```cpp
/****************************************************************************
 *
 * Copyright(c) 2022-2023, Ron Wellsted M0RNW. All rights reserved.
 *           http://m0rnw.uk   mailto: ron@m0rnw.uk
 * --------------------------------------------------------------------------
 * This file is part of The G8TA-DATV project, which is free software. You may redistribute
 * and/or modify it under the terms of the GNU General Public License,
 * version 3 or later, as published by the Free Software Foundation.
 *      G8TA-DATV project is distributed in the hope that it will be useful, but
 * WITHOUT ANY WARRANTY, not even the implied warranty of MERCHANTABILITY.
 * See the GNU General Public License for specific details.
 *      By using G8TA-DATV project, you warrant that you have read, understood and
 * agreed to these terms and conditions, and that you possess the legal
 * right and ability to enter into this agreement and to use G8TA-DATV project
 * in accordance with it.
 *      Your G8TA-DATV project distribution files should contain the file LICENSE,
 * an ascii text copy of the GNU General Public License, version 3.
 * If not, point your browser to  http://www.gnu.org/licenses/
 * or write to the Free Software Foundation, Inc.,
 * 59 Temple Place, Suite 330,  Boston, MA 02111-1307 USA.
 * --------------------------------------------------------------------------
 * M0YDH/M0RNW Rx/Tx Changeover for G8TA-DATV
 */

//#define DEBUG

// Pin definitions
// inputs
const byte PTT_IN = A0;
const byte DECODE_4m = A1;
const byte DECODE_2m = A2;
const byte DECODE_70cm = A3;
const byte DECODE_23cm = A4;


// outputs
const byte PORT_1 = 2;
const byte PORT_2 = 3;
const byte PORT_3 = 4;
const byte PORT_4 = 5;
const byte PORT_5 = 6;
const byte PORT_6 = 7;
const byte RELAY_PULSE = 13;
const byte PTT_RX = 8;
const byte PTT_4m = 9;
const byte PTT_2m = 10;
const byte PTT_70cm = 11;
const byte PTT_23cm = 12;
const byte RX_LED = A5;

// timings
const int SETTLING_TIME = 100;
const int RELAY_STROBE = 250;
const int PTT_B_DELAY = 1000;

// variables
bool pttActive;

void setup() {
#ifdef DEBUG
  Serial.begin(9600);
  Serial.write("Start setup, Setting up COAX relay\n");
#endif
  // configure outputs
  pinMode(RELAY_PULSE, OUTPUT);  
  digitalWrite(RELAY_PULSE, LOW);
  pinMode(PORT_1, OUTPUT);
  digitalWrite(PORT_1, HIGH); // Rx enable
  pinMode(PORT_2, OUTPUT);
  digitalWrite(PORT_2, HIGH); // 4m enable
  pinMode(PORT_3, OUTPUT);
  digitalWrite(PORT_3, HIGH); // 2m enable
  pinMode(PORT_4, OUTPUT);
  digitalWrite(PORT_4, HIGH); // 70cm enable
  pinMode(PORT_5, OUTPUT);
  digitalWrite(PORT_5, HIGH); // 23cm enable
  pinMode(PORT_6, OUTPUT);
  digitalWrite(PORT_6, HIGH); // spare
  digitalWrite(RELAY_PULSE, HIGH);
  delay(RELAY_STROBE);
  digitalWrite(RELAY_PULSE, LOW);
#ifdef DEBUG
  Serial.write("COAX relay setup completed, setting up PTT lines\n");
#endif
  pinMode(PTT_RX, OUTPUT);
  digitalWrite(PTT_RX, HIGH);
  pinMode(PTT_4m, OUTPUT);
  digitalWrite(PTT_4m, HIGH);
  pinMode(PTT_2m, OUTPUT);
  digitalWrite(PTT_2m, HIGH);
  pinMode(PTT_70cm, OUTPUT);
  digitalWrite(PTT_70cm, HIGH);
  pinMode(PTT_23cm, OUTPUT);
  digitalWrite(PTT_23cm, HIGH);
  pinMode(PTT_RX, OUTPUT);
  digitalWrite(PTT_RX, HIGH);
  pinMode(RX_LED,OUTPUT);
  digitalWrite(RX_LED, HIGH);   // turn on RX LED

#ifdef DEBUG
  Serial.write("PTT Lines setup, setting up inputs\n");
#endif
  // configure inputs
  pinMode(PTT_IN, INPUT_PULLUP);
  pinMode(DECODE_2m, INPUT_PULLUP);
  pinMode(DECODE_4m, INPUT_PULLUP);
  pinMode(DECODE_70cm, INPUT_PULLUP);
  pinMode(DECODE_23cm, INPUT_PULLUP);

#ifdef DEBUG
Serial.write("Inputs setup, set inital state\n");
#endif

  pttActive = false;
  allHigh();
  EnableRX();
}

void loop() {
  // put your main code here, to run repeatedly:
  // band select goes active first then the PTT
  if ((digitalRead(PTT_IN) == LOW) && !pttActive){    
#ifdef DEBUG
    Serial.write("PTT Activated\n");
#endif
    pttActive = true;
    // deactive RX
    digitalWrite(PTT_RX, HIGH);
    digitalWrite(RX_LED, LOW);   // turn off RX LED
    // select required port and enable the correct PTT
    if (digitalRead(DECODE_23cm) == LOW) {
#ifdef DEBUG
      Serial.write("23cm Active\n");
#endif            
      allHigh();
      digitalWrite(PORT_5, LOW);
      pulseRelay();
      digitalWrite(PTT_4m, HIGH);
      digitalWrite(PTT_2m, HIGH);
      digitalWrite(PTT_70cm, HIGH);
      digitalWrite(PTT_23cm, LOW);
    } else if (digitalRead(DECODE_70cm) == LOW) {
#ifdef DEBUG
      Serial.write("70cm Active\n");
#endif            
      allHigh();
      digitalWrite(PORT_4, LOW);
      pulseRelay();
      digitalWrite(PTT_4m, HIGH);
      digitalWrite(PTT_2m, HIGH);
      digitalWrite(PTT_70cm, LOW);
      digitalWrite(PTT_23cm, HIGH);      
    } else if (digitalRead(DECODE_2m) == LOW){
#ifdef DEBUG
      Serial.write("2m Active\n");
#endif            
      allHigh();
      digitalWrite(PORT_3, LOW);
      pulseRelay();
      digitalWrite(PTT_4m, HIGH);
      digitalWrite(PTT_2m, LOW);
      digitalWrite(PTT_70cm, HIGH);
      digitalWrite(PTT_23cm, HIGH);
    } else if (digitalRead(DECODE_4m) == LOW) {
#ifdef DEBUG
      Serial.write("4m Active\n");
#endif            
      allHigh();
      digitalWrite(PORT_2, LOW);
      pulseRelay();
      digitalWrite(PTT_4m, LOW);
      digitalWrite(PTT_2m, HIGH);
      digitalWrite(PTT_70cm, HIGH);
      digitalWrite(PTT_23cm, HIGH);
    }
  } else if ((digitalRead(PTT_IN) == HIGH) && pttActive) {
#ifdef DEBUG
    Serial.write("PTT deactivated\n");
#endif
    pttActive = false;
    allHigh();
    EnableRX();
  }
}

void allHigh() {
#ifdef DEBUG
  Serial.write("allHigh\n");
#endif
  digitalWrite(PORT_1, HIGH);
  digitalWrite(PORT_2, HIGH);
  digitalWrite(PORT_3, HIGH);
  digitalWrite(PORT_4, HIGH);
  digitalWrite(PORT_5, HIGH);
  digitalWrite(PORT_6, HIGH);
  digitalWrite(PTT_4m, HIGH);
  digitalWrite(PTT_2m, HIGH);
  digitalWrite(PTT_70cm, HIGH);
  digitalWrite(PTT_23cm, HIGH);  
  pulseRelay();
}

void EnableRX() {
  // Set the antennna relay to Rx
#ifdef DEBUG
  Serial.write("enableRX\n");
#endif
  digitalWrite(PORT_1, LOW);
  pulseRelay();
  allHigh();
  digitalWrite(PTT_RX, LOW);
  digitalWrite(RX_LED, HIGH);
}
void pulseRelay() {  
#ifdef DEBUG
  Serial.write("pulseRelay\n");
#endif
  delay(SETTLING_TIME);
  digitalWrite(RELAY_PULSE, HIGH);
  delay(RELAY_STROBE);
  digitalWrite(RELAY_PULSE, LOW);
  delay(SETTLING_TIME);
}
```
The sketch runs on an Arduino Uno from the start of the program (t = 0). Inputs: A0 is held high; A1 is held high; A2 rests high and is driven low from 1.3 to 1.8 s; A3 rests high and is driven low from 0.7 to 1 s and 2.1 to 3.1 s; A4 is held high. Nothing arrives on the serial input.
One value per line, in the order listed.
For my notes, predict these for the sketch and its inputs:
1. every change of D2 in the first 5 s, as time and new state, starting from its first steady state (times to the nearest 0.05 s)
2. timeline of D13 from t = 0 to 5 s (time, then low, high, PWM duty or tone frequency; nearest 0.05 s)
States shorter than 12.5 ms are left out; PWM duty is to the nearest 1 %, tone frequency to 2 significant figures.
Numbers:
0 s high; 0.7 s low; 1.15 s high
0 s high; 0.25 s low; 0.35 s high; 0.6 s low; 0.8 s high; 1.05 s low; 1.25 s high; 1.5 s low
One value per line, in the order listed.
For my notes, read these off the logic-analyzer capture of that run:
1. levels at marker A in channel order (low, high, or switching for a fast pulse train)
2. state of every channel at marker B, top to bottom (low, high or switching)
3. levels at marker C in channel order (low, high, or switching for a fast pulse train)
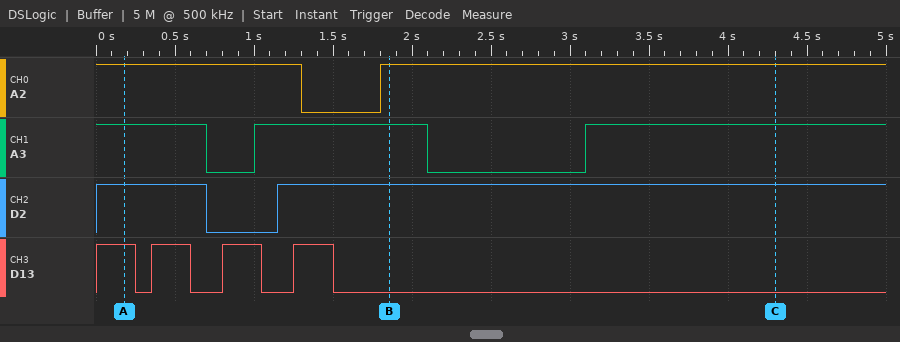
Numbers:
A2 high, A3 high, D2 high, D13 high
A2 high, A3 high, D2 high, D13 low
A2 high, A3 high, D2 high, D13 low
